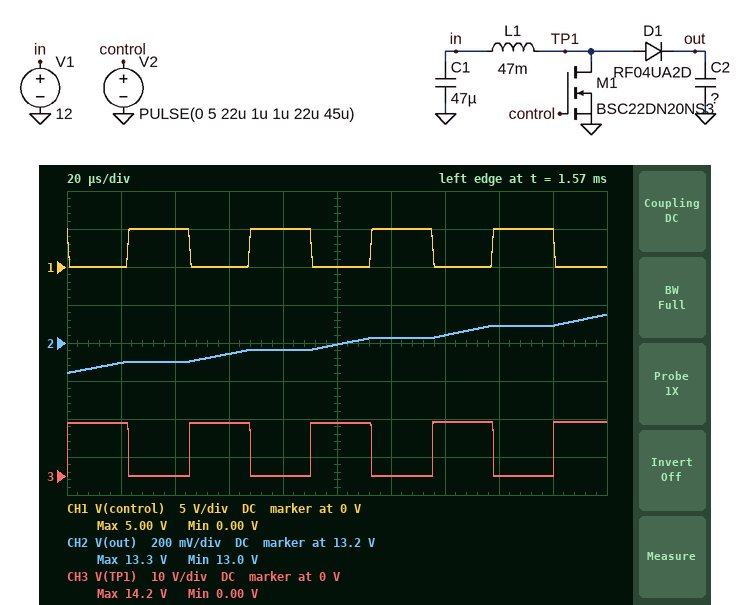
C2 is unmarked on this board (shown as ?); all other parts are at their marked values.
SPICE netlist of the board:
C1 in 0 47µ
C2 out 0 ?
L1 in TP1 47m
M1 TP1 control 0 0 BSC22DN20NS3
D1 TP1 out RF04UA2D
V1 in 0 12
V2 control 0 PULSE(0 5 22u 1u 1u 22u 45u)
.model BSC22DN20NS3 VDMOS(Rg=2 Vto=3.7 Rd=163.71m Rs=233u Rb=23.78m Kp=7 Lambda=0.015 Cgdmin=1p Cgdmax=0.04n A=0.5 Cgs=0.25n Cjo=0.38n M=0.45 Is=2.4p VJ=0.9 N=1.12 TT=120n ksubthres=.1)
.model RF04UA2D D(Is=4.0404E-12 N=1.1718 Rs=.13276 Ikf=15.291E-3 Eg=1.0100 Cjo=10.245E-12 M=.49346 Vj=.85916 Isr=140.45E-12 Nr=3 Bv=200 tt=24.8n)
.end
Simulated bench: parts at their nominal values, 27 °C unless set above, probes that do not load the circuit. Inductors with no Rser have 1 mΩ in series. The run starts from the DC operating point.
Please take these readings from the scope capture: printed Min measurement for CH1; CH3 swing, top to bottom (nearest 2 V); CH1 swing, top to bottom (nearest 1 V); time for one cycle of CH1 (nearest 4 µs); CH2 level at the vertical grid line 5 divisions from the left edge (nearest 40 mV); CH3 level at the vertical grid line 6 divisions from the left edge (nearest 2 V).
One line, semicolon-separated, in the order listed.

0.00 V; 14 V; 5 V; 44 µs; 13.20 V; 0 V
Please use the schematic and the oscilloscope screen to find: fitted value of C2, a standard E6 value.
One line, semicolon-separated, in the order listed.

68 µF
